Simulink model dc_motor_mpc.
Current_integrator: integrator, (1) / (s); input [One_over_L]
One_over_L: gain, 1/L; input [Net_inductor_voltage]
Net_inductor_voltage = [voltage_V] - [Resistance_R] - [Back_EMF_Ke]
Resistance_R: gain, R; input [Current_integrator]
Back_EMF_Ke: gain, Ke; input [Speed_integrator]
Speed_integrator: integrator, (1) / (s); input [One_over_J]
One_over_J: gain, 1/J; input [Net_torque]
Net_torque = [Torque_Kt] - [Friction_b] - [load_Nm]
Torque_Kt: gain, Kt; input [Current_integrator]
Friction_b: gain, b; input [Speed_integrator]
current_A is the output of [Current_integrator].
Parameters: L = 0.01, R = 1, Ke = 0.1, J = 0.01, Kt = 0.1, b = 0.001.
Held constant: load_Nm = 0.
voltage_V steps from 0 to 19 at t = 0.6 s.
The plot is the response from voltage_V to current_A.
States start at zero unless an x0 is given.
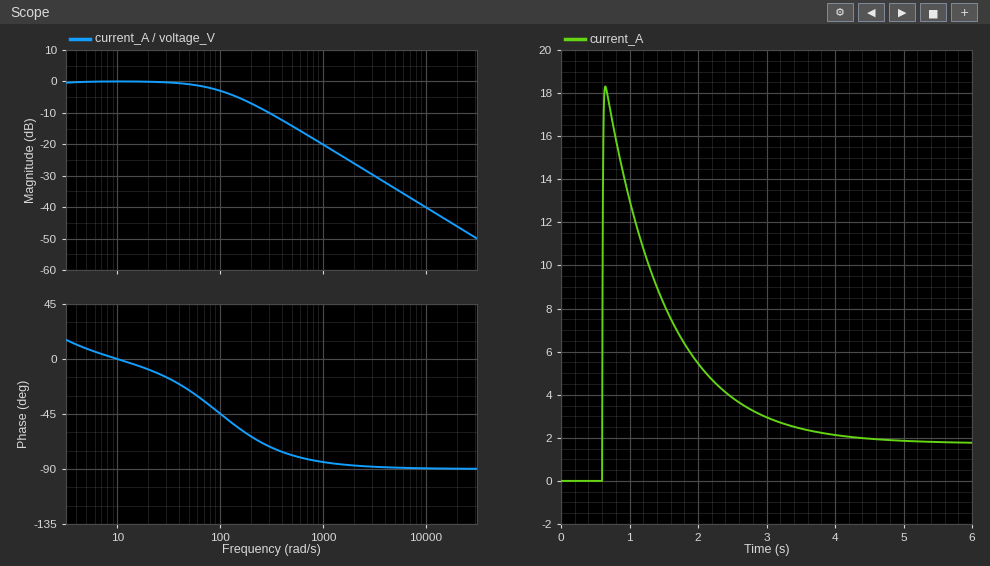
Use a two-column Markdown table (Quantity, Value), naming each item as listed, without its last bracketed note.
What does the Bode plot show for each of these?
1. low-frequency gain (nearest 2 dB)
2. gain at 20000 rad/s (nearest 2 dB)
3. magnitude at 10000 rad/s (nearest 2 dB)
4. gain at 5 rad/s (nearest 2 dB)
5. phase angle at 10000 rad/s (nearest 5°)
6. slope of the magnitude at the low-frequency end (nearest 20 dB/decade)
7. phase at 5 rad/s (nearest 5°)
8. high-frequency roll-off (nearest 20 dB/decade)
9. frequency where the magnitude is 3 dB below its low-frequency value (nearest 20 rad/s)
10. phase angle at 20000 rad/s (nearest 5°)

| Quantity | Value |
|---|---|
| low-frequency gain | 0 dB |
| gain at 20000 rad/s | -46 dB |
| magnitude at 10000 rad/s | -40 dB |
| gain at 5 rad/s | 0 dB |
| phase angle at 10000 rad/s | -90° |
| slope of the magnitude at the low-frequency end | 0 dB/decade |
| phase at 5 rad/s | 10° |
| high-frequency roll-off | -20 dB/decade |
| frequency where the magnitude is 3 dB below its low-frequency value | 100 rad/s |
| phase angle at 20000 rad/s | -90° |
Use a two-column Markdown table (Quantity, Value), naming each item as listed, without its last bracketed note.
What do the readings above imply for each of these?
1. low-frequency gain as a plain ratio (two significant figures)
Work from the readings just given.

| Quantity | Value |
|---|---|
| low-frequency gain as a plain ratio | 1.0 |
